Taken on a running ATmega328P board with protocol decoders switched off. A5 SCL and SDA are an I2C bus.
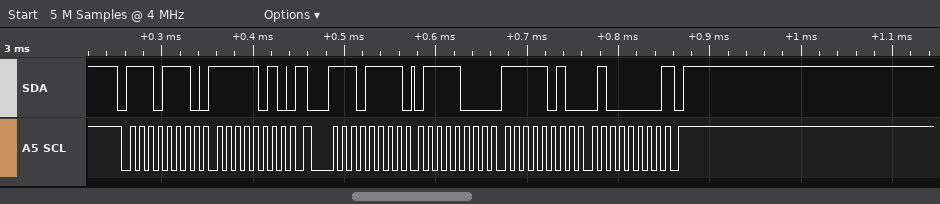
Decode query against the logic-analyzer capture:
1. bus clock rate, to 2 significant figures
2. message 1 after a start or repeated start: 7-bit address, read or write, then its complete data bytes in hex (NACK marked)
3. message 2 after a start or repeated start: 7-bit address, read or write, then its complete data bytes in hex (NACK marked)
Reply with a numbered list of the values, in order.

1. 100 kHz
2. 0x77 write: FA
3. 0x77 read: 78 FA 40 NACK
